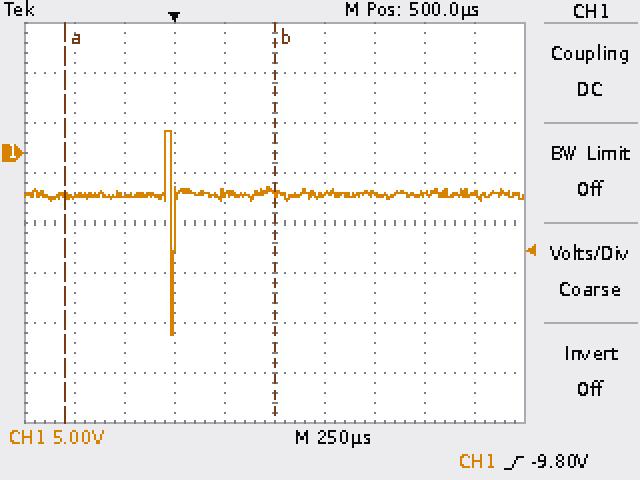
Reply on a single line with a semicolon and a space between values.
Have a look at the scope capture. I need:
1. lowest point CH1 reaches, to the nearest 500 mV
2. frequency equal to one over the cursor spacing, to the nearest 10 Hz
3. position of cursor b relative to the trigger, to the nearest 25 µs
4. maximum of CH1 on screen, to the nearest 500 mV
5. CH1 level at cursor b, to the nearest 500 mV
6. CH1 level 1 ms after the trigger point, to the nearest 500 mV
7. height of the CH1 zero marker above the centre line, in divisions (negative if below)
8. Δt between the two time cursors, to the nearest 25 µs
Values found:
-18.0 V; 950 Hz; +500 µs; 2.0 V; -4.0 V; -4.0 V; +1.4 div; 1.050 ms
